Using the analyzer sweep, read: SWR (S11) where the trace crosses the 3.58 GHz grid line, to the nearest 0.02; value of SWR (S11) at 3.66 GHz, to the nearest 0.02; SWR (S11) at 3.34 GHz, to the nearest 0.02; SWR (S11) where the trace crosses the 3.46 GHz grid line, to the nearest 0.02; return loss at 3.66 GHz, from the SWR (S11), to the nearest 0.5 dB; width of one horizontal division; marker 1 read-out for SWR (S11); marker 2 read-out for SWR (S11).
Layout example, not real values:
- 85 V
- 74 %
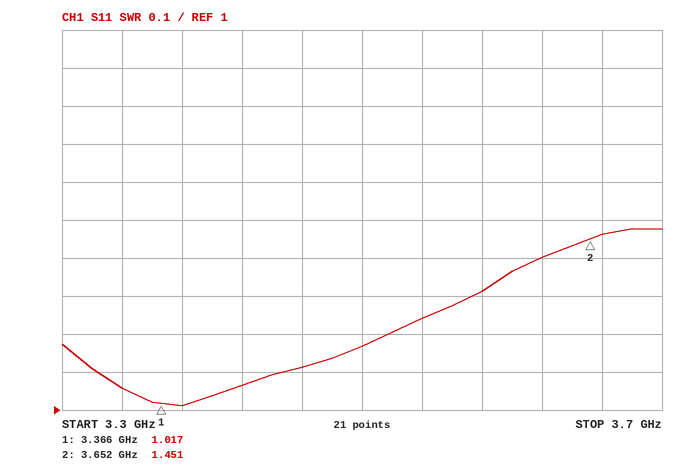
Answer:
- 1.32
- 1.46
- 1.06
- 1.12
- 14.5 dB
- 40 MHz
- 1.017
- 1.451
